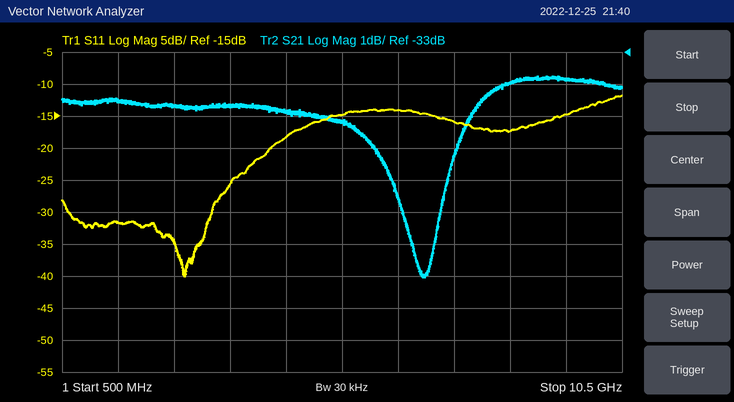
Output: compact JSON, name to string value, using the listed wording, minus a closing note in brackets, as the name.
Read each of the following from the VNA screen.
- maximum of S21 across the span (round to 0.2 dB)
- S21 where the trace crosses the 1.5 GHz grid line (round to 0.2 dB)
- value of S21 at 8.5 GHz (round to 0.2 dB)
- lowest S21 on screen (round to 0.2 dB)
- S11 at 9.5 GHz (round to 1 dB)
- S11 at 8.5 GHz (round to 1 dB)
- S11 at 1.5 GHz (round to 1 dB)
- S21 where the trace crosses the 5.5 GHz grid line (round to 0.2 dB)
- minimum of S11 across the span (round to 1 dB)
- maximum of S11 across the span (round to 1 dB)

{"maximum of S21 across the span": "-33.8 dB", "S21 where the trace crosses the 1.5 GHz grid line": "-34.6 dB", "value of S21 at 8.5 GHz": "-34.0 dB", "lowest S21 on screen": "-40.0 dB", "S11 at 9.5 GHz": "-15 dB", "S11 at 8.5 GHz": "-17 dB", "S11 at 1.5 GHz": "-32 dB", "S21 where the trace crosses the 5.5 GHz grid line": "-35.2 dB", "minimum of S11 across the span": "-40 dB", "maximum of S11 across the span": "-12 dB"}
